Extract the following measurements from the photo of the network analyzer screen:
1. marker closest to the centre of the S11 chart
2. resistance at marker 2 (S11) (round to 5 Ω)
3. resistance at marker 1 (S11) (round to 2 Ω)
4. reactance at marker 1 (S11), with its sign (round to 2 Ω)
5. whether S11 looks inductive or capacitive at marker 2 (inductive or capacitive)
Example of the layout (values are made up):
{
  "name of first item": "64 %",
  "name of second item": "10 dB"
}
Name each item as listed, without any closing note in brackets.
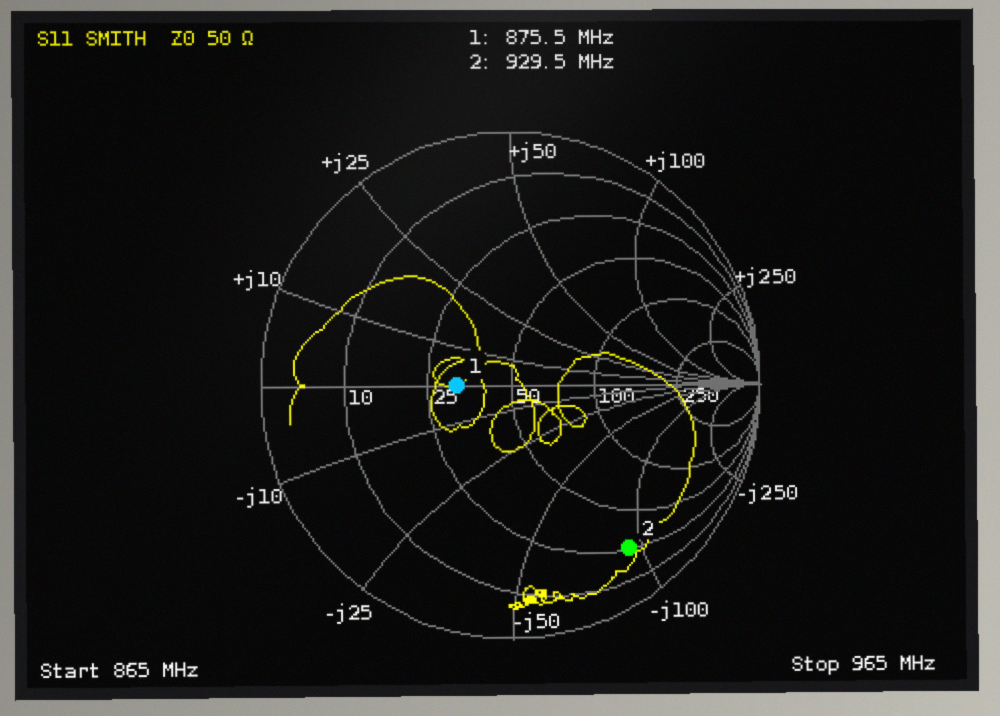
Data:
{
  "marker closest to the centre of the S11 chart": "marker 1",
  "resistance at marker 2 (S11)": "25 Ω",
  "resistance at marker 1 (S11)": "32 Ω",
  "reactance at marker 1 (S11), with its sign": "0 Ω",
  "whether S11 looks inductive or capacitive at marker 2": "capacitive"
}
